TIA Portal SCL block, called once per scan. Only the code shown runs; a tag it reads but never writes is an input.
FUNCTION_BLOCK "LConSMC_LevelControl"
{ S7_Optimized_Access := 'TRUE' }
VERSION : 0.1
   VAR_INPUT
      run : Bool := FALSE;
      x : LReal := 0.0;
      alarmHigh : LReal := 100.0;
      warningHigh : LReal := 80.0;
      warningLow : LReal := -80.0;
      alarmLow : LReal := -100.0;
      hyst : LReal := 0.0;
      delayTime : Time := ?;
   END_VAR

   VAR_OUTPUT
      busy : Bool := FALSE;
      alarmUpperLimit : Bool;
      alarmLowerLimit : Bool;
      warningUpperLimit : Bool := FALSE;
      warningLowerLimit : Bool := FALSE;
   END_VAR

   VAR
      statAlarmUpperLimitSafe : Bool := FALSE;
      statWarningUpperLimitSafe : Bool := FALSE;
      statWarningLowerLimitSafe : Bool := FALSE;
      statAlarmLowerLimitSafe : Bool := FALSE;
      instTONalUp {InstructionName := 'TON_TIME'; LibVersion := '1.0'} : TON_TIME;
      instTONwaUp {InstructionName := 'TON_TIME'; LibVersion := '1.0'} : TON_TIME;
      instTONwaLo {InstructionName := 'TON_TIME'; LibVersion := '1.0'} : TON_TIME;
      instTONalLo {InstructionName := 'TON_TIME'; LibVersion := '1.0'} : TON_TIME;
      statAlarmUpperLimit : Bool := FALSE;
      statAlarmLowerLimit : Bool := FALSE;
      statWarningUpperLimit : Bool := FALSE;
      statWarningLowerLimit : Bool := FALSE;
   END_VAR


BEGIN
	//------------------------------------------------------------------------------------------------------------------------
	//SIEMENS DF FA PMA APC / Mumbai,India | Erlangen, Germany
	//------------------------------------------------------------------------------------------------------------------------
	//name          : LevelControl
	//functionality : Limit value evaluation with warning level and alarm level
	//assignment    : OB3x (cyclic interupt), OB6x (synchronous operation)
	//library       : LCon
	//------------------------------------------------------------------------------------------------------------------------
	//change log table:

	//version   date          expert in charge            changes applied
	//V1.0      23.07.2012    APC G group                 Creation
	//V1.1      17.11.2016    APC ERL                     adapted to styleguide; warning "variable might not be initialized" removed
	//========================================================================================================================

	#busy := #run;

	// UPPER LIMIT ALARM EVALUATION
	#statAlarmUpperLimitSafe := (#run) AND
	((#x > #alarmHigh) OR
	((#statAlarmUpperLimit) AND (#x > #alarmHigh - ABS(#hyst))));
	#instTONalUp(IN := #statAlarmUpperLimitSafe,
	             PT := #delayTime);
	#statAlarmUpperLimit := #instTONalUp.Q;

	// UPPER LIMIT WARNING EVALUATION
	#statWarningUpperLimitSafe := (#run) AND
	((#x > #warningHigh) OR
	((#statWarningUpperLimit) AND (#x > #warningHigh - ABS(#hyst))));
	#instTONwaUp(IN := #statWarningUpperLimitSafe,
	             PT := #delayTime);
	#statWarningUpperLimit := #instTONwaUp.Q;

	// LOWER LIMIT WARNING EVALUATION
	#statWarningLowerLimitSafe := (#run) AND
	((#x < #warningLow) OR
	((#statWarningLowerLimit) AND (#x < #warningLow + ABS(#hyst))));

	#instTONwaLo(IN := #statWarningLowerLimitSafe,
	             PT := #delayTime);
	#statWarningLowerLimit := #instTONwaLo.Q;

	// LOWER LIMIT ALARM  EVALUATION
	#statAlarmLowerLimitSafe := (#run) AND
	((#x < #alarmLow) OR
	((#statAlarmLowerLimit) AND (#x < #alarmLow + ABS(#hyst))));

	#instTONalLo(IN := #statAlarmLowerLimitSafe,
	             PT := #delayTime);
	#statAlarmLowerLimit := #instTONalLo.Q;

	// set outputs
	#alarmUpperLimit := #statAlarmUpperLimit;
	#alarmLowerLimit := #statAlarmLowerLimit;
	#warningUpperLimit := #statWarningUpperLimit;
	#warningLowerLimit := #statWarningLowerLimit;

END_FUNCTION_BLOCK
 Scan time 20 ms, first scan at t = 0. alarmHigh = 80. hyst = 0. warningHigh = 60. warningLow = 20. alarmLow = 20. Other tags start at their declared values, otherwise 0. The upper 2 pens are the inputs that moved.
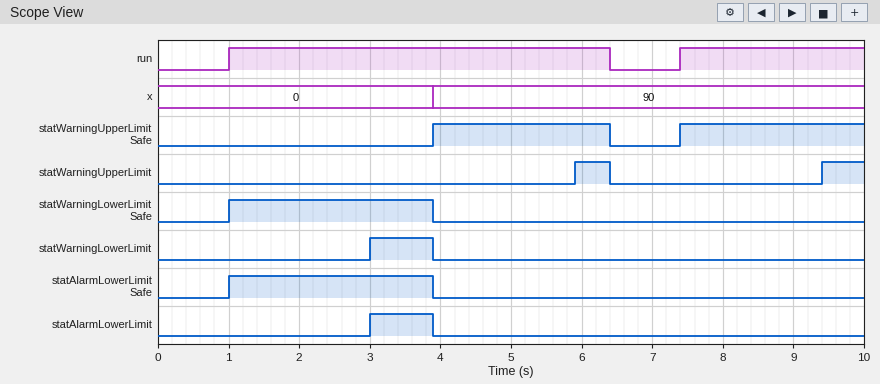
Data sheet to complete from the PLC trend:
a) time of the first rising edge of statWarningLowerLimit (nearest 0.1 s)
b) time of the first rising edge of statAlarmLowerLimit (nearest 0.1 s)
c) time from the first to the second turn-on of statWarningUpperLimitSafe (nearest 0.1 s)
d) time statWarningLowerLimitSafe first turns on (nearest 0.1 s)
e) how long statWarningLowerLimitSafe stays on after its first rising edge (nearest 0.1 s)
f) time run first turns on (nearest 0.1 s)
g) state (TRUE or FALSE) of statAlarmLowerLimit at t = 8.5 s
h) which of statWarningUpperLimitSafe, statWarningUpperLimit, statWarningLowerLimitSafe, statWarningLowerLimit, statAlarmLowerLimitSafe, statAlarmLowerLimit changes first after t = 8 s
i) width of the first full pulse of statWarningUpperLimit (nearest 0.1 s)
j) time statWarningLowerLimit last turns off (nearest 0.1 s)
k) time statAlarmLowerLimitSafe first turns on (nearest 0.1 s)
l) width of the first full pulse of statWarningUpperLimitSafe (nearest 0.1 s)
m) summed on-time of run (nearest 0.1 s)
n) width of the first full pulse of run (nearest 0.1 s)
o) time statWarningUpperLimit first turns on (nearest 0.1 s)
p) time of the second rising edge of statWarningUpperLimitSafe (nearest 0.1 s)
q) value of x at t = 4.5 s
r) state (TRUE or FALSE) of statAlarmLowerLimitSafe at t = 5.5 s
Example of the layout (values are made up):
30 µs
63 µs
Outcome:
3.0 s
3.0 s
3.5 s
1.0 s
2.9 s
1.0 s
FALSE
statWarningUpperLimit
0.5 s
3.9 s
1.0 s
2.5 s
8.0 s
5.4 s
5.9 s
7.4 s
90
FALSE
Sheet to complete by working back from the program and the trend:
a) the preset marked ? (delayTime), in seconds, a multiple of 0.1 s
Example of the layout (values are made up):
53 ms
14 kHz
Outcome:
2.0 s
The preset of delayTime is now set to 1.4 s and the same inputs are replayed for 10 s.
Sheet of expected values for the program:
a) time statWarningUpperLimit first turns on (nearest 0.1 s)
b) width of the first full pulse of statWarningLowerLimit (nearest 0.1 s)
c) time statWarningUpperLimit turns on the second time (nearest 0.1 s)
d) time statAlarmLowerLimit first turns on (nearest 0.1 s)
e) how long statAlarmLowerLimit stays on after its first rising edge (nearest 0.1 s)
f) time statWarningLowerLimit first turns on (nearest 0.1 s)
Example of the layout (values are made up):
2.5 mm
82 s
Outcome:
5.3 s
1.5 s
8.8 s
2.4 s
1.5 s
2.4 s
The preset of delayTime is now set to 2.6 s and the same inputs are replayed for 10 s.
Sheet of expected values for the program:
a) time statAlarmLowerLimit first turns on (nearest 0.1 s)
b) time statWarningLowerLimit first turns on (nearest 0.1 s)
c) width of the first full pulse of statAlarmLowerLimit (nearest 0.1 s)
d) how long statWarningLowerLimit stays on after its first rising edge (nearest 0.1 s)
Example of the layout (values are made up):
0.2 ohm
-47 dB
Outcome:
3.6 s
3.6 s
0.3 s
0.3 s
